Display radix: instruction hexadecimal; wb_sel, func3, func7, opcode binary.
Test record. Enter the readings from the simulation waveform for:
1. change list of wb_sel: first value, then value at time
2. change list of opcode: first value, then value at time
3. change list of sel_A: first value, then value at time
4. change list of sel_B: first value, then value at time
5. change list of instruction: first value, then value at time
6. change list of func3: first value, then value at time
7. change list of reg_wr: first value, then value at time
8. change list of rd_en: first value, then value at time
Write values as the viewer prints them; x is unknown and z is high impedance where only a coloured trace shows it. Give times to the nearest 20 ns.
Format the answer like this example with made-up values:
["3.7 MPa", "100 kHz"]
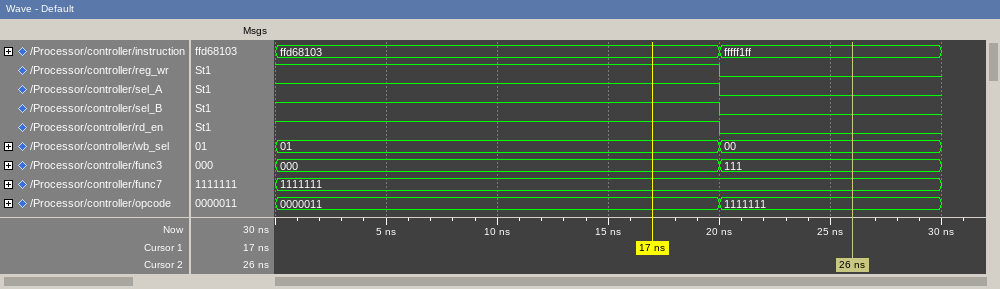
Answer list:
["01, 00 at 20 ns", "0000011, 1111111 at 20 ns", "1, 0 at 20 ns", "1, 0 at 20 ns", "ffd68103, fffff1ff at 20 ns", "000, 111 at 20 ns", "1, 0 at 20 ns", "1, 0 at 20 ns"]
